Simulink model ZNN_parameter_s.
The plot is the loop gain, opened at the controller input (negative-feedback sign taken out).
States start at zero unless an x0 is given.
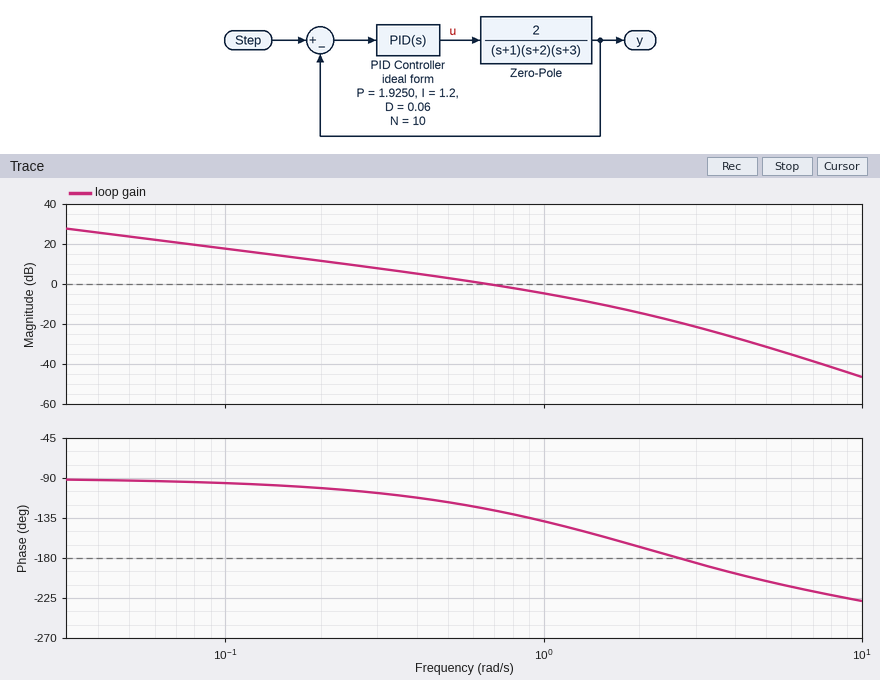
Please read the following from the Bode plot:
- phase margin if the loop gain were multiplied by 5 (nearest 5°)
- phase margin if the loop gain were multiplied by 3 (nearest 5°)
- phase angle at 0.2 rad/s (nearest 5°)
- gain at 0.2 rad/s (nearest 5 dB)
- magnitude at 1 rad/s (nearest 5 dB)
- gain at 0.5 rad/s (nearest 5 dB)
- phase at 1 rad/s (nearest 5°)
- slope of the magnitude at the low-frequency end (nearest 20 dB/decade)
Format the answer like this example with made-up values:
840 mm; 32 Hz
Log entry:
15°; 25°; -100°; 10 dB; -5 dB; 5 dB; -140°; -20 dB/decade
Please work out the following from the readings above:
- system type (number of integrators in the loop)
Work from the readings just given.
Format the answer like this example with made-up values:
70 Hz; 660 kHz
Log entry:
1
